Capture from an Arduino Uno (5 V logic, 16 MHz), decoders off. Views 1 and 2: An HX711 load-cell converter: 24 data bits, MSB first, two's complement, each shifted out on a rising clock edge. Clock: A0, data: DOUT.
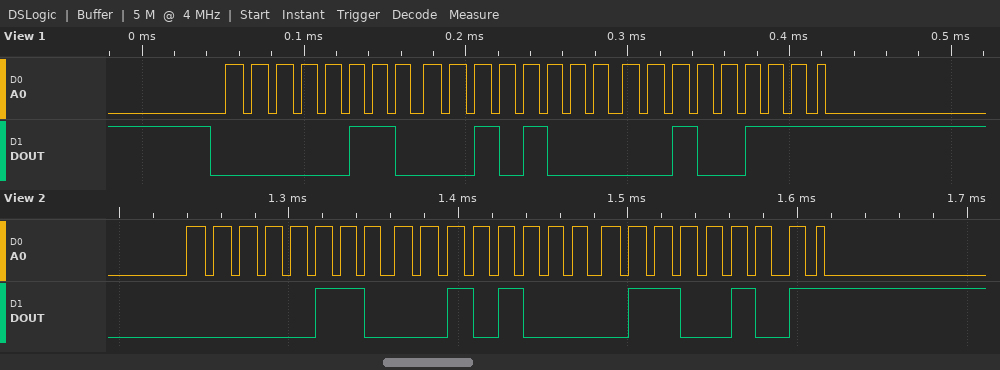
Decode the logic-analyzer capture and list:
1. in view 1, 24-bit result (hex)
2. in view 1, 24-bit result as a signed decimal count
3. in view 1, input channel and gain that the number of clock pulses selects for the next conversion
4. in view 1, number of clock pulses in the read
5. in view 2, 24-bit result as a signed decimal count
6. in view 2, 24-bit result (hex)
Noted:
0x062827
403495
channel A, gain 128
25
403557
0x062865
